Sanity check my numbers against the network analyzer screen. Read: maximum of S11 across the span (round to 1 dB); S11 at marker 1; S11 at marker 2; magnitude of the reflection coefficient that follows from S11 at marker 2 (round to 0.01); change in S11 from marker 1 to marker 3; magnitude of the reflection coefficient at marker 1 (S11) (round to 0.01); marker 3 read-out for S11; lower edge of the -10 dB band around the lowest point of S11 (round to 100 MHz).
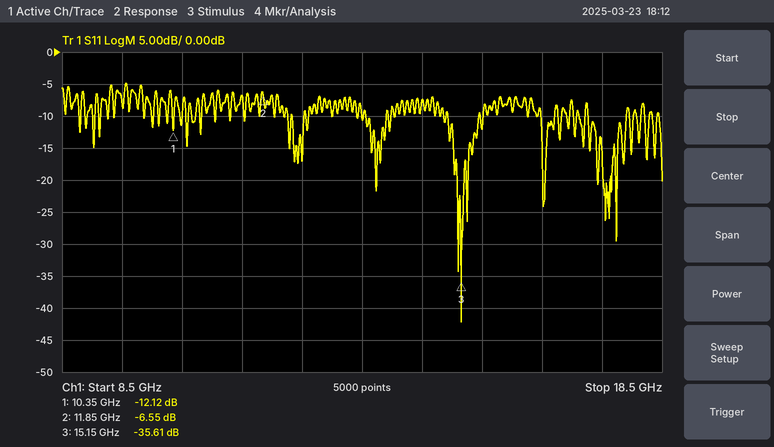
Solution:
-5 dB
-12.12 dB
-6.55 dB
0.47
-23.49 dB
0.25
-35.61 dB
14.9 GHz
